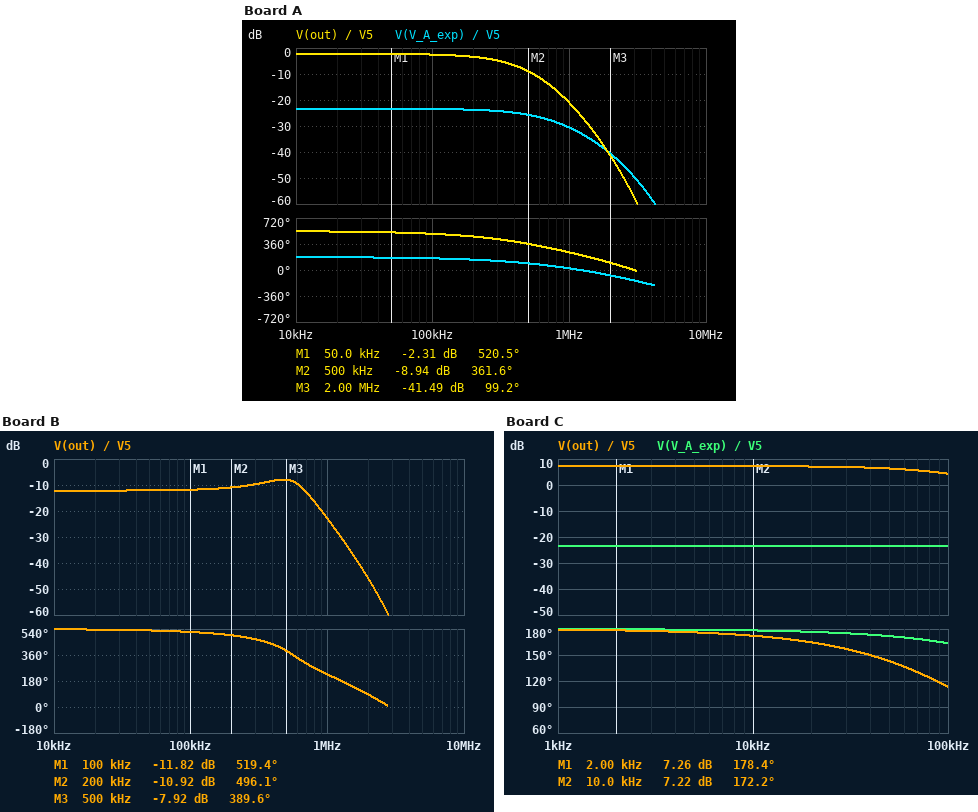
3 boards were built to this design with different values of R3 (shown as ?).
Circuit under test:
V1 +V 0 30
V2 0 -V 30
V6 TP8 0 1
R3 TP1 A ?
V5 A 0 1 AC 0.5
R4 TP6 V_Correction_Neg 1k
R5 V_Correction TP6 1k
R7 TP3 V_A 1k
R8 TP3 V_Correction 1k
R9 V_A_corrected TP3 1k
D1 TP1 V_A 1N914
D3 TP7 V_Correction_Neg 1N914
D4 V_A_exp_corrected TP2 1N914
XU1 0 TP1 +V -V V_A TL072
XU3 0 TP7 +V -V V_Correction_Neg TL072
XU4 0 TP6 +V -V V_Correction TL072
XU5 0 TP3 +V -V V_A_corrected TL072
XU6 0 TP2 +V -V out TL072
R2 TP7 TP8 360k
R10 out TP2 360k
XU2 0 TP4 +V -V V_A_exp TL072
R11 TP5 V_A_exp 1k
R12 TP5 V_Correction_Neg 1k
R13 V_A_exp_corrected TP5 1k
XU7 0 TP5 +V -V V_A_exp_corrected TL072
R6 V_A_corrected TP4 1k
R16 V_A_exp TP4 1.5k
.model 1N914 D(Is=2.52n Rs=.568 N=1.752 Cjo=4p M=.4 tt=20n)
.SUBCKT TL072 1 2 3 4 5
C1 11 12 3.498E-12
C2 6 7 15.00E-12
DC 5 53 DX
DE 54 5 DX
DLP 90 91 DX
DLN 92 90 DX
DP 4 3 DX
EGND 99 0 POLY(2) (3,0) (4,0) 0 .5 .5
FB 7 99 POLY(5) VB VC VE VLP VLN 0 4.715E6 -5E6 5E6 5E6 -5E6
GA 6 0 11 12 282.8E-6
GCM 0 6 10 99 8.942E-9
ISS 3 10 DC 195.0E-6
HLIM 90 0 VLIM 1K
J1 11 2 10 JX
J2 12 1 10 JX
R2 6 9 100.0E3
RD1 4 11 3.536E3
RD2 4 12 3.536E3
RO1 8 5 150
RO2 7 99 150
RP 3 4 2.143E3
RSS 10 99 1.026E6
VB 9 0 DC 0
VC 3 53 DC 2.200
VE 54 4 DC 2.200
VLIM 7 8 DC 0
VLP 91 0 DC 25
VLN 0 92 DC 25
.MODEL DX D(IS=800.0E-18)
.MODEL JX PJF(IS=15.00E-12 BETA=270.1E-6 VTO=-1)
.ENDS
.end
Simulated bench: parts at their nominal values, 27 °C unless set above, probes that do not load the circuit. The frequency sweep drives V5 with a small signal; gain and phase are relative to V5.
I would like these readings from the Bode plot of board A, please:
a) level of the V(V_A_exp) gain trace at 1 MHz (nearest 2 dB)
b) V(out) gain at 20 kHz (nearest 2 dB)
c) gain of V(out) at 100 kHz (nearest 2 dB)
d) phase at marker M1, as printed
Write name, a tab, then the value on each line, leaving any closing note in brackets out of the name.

level of the V(V_A_exp) gain trace at 1 MHz	-30 dB
V(out) gain at 20 kHz	-2 dB
gain of V(out) at 100 kHz	-2 dB
phase at marker M1, as printed	520.5 deg
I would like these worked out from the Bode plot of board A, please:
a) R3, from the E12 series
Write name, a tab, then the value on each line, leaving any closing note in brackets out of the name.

R3, from the E12 series	560 kΩ
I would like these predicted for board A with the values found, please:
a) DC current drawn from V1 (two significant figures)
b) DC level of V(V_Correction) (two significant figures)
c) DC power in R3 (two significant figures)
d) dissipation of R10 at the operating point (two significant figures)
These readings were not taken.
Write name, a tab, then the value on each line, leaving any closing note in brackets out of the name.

DC current drawn from V1	200 mA
DC level of V(V_Correction)	320 mV
DC power in R3	1.8 µW
dissipation of R10 at the operating point	740 nW
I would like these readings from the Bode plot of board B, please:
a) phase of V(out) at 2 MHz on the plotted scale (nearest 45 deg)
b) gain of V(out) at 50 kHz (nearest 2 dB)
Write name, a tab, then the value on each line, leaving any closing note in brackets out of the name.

phase of V(out) at 2 MHz on the plotted scale	90 deg
gain of V(out) at 50 kHz	-12 dB
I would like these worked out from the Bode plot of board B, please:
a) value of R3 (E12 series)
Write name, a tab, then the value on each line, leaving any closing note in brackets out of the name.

value of R3	1.2 MΩ
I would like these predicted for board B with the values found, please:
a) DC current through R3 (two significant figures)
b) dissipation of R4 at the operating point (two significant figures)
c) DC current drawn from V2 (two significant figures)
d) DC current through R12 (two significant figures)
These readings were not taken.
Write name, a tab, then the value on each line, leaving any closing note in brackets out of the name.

DC current through R3	830 nA
dissipation of R4 at the operating point	100 µW
DC current drawn from V2	200 mA
DC current through R12	320 µA
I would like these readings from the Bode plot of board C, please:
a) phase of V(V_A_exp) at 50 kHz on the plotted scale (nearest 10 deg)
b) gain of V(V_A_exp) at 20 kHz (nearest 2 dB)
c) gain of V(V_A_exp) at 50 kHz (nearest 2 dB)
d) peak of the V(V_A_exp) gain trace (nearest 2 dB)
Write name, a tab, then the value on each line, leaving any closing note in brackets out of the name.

phase of V(V_A_exp) at 50 kHz on the plotted scale	170 deg
gain of V(V_A_exp) at 20 kHz	-24 dB
gain of V(V_A_exp) at 50 kHz	-24 dB
peak of the V(V_A_exp) gain trace	-24 dB
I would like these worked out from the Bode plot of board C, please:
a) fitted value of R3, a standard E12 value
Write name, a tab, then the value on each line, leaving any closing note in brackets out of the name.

fitted value of R3, a standard E12 value	270 kΩ
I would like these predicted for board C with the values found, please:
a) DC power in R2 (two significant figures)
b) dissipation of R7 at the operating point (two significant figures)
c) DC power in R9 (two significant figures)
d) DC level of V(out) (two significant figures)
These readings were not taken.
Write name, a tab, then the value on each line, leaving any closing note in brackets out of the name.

DC power in R2	2.8 µW
dissipation of R7 at the operating point	110 µW
DC power in R9	170 nW
DC level of V(out)	-1.5 V
